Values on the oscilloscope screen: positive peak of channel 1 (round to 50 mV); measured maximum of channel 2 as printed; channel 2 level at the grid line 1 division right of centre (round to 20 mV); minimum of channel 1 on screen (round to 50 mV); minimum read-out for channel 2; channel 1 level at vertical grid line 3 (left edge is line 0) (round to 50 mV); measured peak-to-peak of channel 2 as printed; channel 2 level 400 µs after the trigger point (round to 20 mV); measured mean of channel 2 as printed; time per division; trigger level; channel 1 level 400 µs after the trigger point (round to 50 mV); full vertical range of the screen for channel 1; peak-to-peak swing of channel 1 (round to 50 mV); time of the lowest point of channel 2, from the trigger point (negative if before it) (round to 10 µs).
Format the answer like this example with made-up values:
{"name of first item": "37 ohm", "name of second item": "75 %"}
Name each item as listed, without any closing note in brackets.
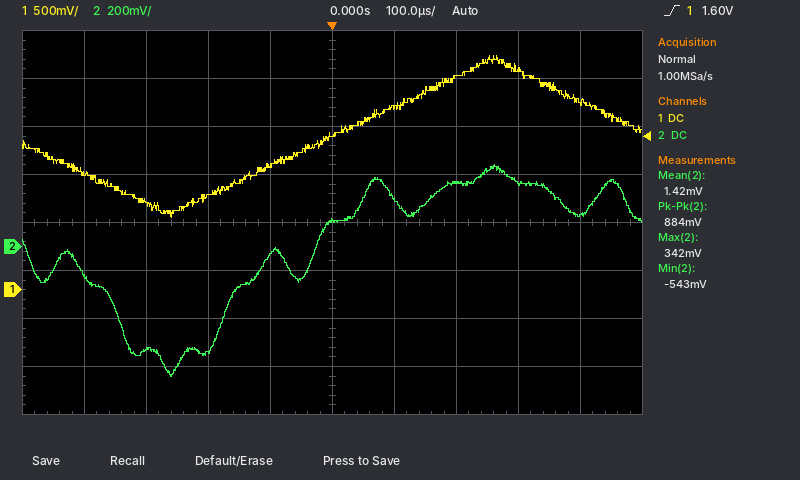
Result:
{"positive peak of channel 1": "2.45 V", "measured maximum of channel 2 as printed": "342 mV", "channel 2 level at the grid line 1 division right of centre": "200 mV", "minimum of channel 1 on screen": "750 mV", "minimum read-out for channel 2": "-543 mV", "channel 1 level at vertical grid line 3 (left edge is line 0)": "950 mV", "measured peak-to-peak of channel 2 as printed": "884 mV", "channel 2 level 400 µs after the trigger point": "140 mV", "measured mean of channel 2 as printed": "1.42 mV", "time per division": "100 µs", "trigger level": "1.60 V", "channel 1 level 400 µs after the trigger point": "1.95 V", "full vertical range of the screen for channel 1": "4 V", "peak-to-peak swing of channel 1": "1.70 V", "time of the lowest point of channel 2, from the trigger point (negative if before it)": "-260 µs"}
